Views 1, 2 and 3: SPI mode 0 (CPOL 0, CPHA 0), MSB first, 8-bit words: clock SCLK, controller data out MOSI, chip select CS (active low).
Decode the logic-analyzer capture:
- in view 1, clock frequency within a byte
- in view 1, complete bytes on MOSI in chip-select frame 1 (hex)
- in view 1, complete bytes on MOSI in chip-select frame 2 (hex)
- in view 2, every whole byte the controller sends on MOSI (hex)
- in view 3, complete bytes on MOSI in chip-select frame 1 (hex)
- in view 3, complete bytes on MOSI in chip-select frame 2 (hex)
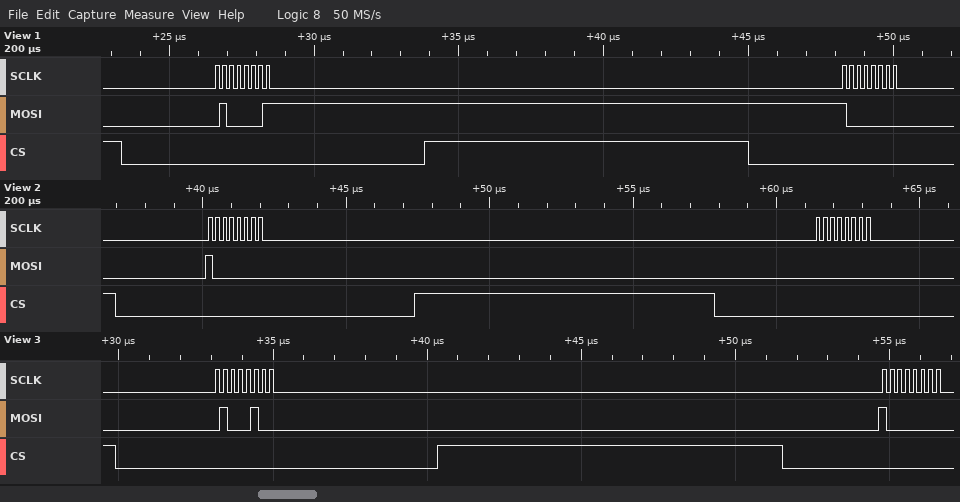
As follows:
4 MHz
41
80
80 00
44
80
